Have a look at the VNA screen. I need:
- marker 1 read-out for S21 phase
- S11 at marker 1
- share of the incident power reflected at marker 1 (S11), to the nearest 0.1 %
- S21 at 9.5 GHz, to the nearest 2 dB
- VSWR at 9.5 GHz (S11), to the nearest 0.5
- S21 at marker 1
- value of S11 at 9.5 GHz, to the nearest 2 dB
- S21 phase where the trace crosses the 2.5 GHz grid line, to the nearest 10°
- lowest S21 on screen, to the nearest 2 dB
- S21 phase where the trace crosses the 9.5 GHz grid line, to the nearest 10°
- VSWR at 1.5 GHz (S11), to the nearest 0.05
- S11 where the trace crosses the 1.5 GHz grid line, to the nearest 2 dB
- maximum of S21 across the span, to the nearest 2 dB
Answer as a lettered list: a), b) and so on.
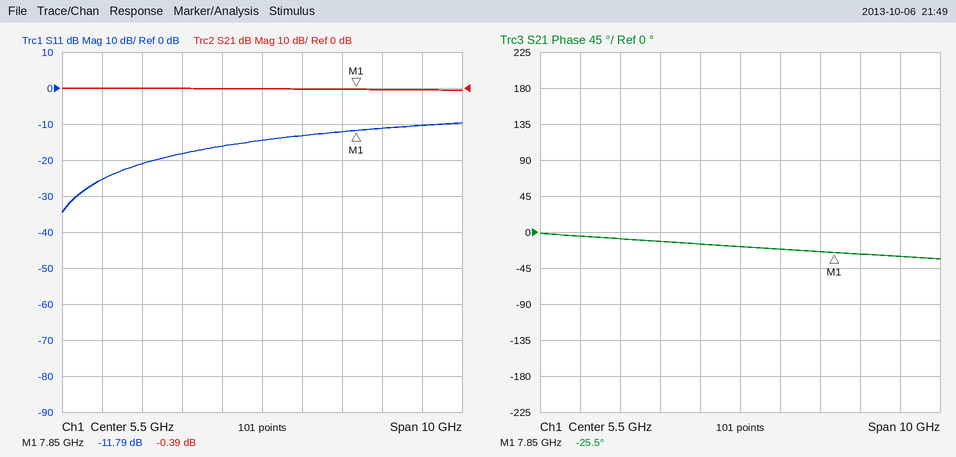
a) -25.5°
b) -11.79 dB
c) 6.6 %
d) 0 dB
e) 2.0
f) -0.39 dB
g) -10 dB
h) -10°
i) 0 dB
j) -30°
k) 1.10
l) -26 dB
m) 0 dB
